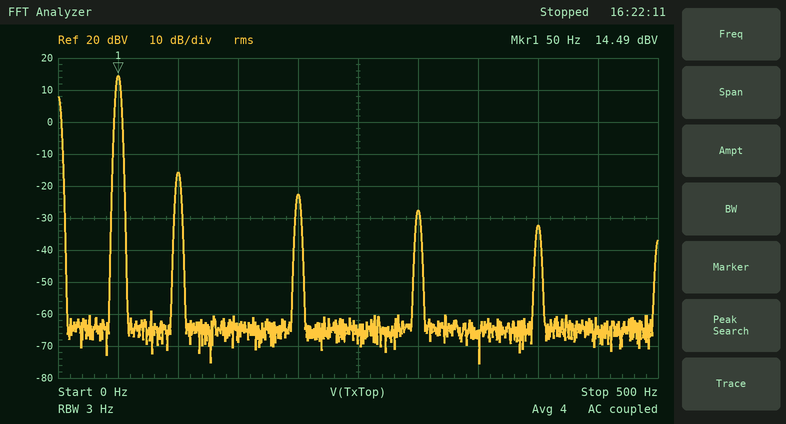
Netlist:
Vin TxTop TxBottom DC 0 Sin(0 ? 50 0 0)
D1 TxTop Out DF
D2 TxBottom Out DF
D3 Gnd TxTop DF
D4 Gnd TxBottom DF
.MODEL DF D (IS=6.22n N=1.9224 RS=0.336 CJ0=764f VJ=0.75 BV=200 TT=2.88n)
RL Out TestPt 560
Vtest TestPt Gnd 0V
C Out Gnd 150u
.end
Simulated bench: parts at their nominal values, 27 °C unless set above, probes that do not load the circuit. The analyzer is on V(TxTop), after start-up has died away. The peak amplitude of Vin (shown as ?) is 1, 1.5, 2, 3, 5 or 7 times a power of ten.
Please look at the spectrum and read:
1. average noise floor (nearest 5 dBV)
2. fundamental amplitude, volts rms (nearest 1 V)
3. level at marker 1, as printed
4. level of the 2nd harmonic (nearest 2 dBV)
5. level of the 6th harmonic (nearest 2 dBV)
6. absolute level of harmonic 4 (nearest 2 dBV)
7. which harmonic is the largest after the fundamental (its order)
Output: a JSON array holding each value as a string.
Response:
["-65 dBV", "5 V", "14.49 dBV", "-16 dBV", "-28 dBV", "-22 dBV", "2"]
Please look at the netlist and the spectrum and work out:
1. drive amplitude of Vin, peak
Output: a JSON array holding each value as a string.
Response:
["15 V"]
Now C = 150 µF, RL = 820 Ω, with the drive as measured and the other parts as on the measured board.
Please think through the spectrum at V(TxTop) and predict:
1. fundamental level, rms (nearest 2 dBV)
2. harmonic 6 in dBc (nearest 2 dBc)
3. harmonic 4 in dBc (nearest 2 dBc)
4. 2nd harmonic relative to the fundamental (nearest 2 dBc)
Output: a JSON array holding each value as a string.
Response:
["14 dBV", "-44 dBc", "-40 dBc", "-34 dBc"]
